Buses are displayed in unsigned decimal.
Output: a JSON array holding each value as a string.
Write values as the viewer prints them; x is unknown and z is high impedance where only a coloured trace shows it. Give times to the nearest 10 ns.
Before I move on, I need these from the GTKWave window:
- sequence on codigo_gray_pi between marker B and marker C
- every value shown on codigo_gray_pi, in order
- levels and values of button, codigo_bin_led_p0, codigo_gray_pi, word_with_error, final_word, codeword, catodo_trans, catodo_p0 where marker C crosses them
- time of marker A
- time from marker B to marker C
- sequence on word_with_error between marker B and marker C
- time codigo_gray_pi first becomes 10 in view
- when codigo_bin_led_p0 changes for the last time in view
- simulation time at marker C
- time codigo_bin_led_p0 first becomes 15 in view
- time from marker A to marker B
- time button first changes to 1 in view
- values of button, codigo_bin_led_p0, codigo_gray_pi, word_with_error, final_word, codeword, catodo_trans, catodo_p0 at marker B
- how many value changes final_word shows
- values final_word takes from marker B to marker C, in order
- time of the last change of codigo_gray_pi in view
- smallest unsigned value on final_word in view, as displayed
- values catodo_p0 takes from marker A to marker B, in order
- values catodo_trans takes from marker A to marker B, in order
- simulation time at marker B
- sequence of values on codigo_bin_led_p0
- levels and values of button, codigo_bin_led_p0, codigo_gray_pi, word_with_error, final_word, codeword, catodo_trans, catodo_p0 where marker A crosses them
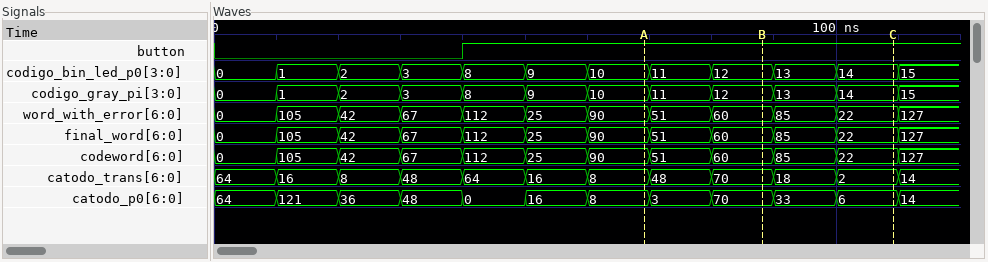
["12, 13, 14", "0, 1, 2, 3, 8, 9, 10, 11, 12, 13, 14, 15", "button=1, codigo_bin_led_p0=14, codigo_gray_pi=14, word_with_error=22, final_word=22, codeword=22, catodo_trans=2, catodo_p0=6", "70 ns", "20 ns", "60, 85, 22", "60 ns", "110 ns", "110 ns", "110 ns", "20 ns", "40 ns", "button=1, codigo_bin_led_p0=12, codigo_gray_pi=12, word_with_error=60, final_word=60, codeword=60, catodo_trans=70, catodo_p0=70", "11", "60, 85, 22", "110 ns", "0", "8, 3, 70", "8, 48, 70", "90 ns", "0, 1, 2, 3, 8, 9, 10, 11, 12, 13, 14, 15", "button=1, codigo_bin_led_p0=10, codigo_gray_pi=10, word_with_error=90, final_word=90, codeword=90, catodo_trans=8, catodo_p0=8"]
